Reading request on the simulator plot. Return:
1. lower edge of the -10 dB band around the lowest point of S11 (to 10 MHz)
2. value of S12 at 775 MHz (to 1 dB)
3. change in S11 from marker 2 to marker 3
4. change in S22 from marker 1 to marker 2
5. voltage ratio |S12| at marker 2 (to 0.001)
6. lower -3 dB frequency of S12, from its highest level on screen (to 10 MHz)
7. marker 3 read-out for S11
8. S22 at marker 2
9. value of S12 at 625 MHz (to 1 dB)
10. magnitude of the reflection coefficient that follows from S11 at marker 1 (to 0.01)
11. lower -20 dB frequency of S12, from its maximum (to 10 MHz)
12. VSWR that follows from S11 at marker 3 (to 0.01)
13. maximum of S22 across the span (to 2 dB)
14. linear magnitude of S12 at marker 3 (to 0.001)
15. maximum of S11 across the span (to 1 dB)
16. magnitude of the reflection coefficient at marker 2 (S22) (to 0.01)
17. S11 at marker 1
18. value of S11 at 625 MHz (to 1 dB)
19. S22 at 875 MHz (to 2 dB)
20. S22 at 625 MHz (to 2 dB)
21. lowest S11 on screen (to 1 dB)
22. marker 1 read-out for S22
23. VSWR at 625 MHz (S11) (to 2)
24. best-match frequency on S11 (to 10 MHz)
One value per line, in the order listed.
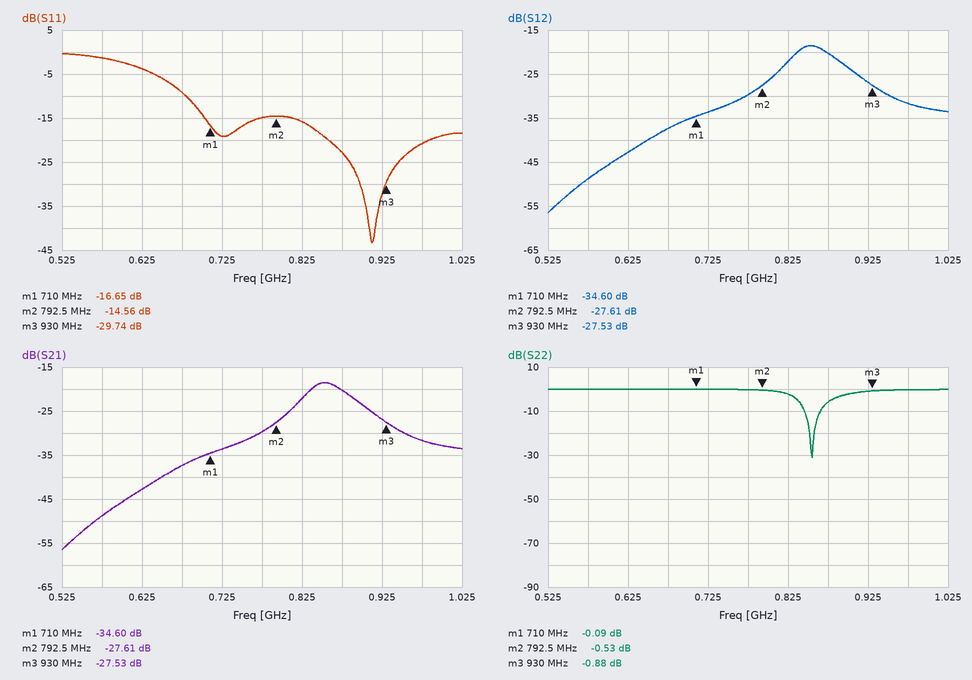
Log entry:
680 MHz
-30 dB
-15.18 dB
-0.44 dB
0.042
830 MHz
-29.74 dB
-0.53 dB
-43 dB
0.15
660 MHz
1.07
0 dB
0.042
0 dB
0.94
-16.65 dB
-4 dB
-6 dB
0 dB
-43 dB
-0.09 dB
4
910 MHz
